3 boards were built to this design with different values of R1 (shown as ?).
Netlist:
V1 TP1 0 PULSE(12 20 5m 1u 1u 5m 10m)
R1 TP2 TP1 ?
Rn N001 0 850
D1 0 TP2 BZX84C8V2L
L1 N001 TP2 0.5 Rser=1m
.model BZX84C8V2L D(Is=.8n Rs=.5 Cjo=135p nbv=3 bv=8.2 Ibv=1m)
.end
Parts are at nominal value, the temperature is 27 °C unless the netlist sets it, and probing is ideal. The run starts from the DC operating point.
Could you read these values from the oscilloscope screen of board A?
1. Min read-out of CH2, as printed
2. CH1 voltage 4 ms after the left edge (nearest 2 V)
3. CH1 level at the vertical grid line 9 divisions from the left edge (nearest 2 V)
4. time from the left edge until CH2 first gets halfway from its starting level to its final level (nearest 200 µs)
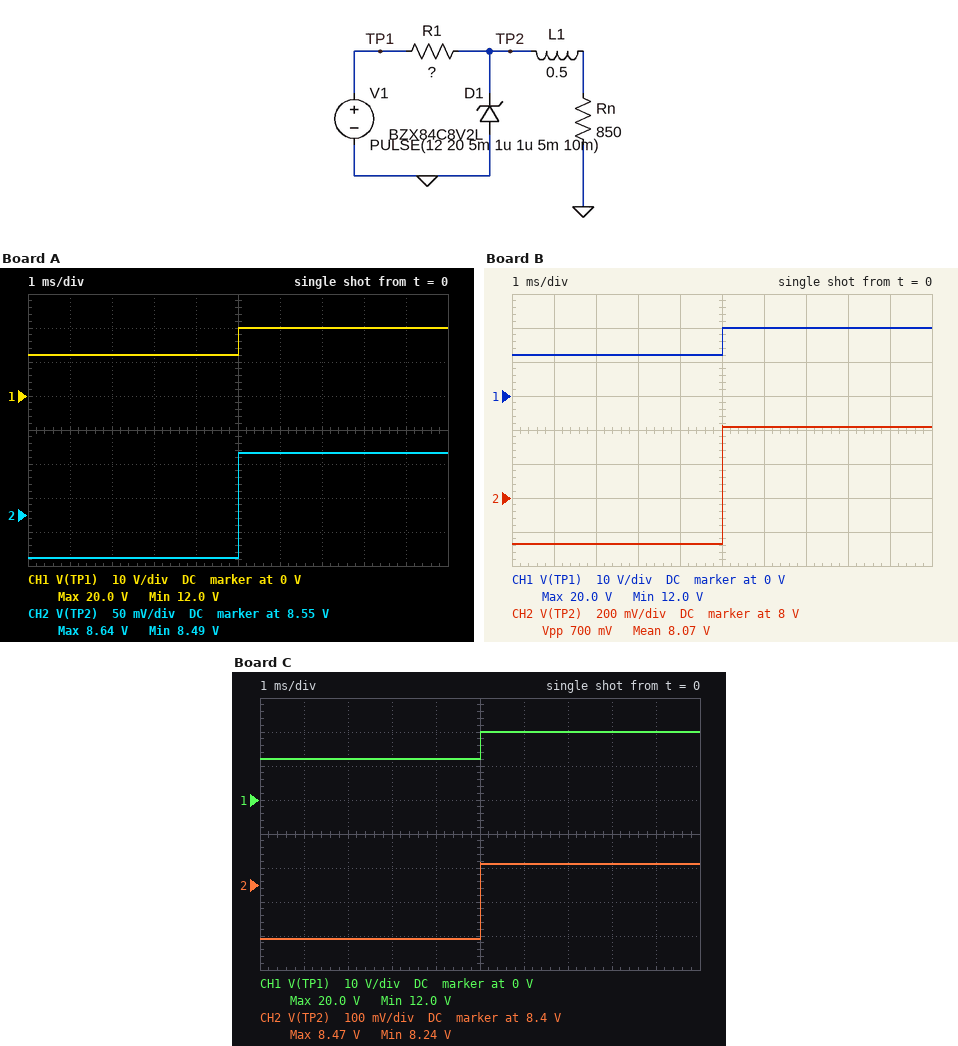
8.49 V
12 V
20 V
5.0 ms
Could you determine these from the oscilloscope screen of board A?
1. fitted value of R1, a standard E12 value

82 Ω
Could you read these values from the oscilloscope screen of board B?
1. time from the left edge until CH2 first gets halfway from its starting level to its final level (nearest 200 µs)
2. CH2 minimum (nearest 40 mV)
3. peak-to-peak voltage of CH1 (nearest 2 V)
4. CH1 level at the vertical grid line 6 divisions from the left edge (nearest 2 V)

5.0 ms
7.72 V
8 V
20 V
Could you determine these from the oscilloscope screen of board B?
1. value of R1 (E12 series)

470 Ω
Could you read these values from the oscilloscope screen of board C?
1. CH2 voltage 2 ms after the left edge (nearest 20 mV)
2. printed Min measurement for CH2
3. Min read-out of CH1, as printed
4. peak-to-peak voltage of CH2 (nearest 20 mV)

8.24 V
8.24 V
12.0 V
220 mV
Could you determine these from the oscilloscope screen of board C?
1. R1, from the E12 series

330 Ω
